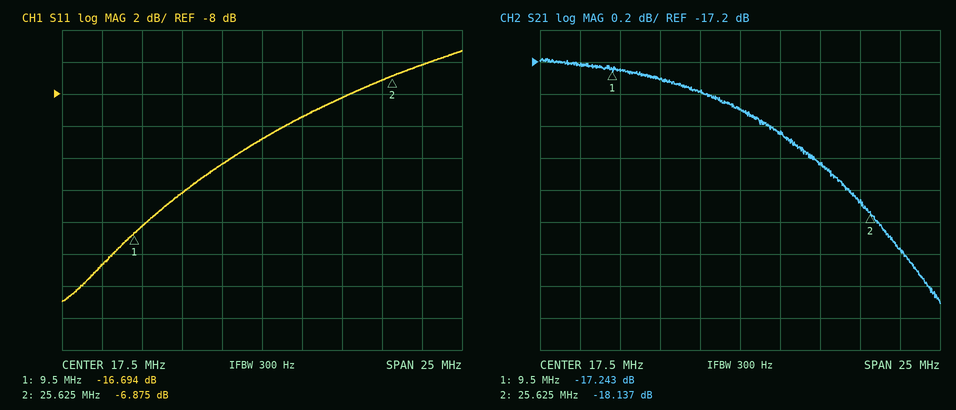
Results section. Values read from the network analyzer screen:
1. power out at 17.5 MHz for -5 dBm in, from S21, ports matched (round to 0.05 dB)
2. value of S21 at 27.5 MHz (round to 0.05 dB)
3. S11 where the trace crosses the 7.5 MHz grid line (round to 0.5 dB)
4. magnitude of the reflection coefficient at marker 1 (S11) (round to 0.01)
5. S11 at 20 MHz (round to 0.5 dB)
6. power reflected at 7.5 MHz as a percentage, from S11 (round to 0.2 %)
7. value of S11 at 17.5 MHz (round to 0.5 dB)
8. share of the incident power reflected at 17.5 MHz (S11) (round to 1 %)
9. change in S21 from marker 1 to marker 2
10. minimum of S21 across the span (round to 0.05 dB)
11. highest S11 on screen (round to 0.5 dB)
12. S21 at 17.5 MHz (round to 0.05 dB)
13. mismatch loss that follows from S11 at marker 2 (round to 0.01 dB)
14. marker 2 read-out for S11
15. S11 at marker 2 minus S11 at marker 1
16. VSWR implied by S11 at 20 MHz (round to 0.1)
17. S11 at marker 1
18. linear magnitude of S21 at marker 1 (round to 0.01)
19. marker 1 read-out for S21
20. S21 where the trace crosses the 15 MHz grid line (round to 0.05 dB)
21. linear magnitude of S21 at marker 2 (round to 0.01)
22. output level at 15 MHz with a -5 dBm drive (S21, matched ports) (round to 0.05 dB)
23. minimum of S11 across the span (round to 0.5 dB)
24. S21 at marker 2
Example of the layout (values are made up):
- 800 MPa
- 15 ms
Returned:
- -22.50 dBm
- -18.35 dB
- -18.5 dB
- 0.15
- -9.5 dB
- 1.4 %
- -11.0 dB
- 8 %
- -0.894 dB
- -18.70 dB
- -5.5 dB
- -17.50 dB
- 1.00 dB
- -6.875 dB
- 9.819 dB
- 2.0
- -16.694 dB
- 0.14
- -17.243 dB
- -17.40 dB
- 0.12
- -22.40 dBm
- -21.0 dB
- -18.137 dB
